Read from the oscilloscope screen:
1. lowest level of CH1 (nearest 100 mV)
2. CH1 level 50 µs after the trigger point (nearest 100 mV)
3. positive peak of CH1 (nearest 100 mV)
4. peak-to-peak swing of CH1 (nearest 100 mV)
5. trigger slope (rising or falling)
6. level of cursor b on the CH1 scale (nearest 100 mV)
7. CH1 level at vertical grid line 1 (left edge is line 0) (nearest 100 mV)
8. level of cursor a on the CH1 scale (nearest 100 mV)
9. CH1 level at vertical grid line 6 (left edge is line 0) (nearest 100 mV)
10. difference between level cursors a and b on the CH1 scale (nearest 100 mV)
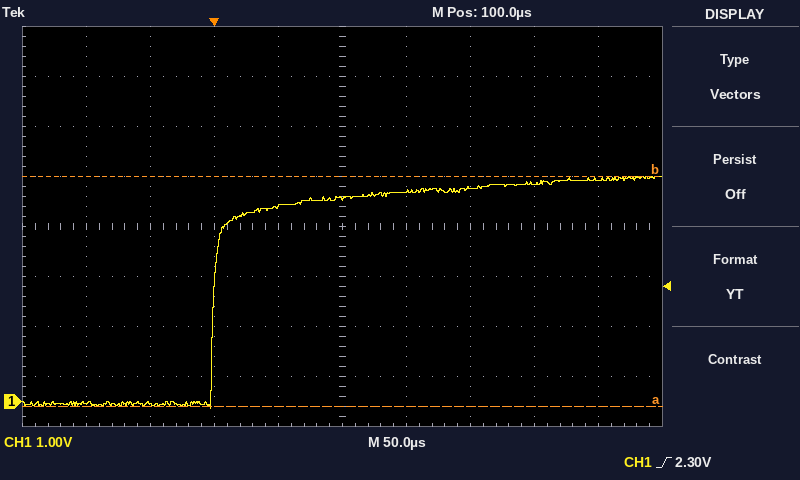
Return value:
-100 mV
3.9 V
4.5 V
4.6 V
rising
4.5 V
0.0 V
-100 mV
4.2 V
4.6 V
